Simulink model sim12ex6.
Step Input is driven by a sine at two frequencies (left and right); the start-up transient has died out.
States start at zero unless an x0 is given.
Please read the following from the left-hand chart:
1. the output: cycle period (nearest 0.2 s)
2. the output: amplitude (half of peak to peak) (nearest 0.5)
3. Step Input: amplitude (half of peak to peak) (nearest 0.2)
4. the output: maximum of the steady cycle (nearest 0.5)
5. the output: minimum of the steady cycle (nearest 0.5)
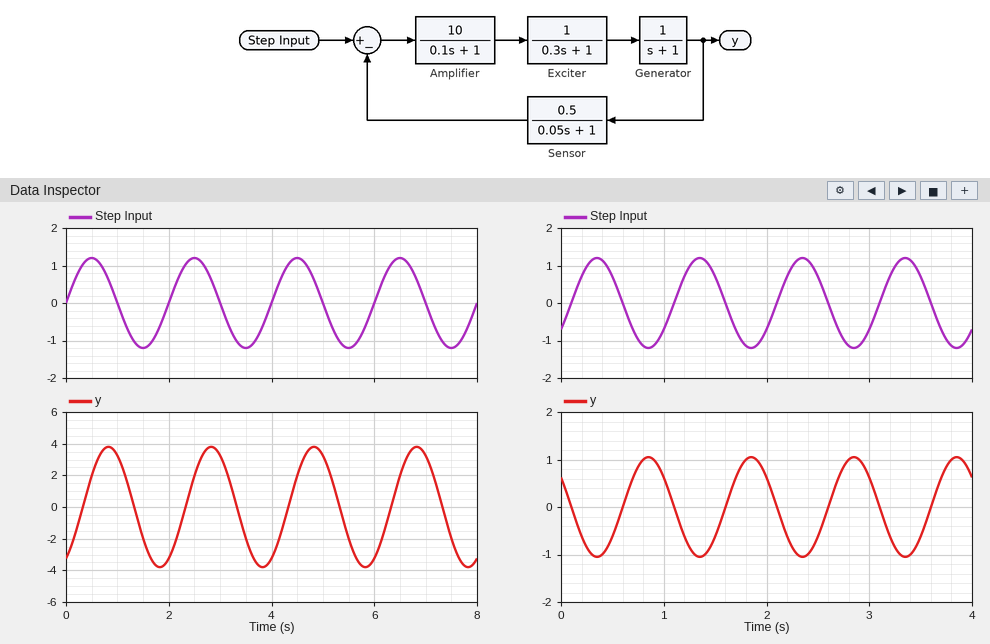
2.0 s
4.0
1.2
4.0
-4.0
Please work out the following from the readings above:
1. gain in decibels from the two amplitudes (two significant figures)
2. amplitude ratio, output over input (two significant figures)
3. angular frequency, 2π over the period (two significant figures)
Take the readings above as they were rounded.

10 dB
3.3
3.1 rad/s
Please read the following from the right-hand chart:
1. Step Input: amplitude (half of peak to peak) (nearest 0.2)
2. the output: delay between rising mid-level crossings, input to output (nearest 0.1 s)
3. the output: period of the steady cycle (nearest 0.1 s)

1.2
0.5 s
1.0 s
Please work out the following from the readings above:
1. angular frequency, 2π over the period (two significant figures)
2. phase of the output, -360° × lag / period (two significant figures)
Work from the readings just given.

6.3 rad/s
-180°
